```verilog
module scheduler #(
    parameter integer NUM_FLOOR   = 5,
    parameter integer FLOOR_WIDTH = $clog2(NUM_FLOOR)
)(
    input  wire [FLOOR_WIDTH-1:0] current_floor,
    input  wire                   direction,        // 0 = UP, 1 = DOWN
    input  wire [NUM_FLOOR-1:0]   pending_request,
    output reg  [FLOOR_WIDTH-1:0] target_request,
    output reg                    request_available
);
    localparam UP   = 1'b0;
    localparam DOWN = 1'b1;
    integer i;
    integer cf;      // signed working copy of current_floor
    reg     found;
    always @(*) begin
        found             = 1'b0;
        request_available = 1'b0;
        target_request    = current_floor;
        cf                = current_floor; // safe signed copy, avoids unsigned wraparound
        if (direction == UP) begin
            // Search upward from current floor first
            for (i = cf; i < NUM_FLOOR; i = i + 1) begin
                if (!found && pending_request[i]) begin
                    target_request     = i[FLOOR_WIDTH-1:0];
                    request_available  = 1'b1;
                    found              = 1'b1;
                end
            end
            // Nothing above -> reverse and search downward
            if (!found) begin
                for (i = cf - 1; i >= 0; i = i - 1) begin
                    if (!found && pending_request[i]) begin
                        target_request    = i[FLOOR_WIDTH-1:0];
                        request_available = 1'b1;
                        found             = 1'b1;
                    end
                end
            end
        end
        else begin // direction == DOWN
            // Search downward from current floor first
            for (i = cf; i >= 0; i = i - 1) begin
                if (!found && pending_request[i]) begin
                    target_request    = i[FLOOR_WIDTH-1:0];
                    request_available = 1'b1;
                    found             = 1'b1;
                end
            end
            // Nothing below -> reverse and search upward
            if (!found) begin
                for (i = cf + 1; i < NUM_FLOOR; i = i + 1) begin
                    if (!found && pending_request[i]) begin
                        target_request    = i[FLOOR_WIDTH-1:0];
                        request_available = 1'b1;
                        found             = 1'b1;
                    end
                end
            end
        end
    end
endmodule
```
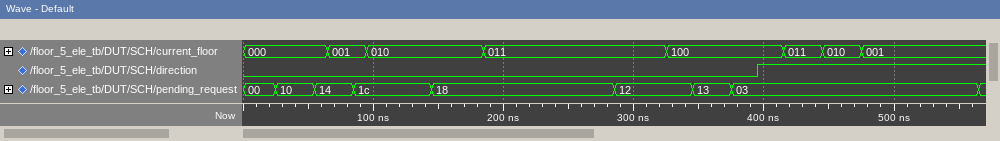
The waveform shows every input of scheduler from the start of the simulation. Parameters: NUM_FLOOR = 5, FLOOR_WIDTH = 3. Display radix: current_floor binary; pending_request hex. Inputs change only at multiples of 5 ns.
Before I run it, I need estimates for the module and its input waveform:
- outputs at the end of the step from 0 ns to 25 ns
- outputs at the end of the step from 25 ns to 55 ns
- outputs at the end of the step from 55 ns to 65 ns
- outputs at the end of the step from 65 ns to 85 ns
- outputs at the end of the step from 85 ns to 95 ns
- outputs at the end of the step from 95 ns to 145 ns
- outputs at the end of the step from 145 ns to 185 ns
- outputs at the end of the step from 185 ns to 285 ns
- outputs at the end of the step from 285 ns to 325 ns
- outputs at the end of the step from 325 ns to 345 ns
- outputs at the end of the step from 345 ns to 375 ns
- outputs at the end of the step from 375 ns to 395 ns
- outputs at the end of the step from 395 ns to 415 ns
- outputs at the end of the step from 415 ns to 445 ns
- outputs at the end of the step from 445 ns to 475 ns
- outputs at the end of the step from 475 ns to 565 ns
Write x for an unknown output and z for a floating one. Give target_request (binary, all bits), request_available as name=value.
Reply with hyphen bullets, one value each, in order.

- target_request=000, request_available=0
- target_request=100, request_available=1
- target_request=010, request_available=1
- target_request=010, request_available=1
- target_request=010, request_available=1
- target_request=010, request_available=1
- target_request=011, request_available=1
- target_request=011, request_available=1
- target_request=100, request_available=1
- target_request=100, request_available=1
- target_request=100, request_available=1
- target_request=001, request_available=1
- target_request=001, request_available=1
- target_request=001, request_available=1
- target_request=001, request_available=1
- target_request=001, request_available=1
